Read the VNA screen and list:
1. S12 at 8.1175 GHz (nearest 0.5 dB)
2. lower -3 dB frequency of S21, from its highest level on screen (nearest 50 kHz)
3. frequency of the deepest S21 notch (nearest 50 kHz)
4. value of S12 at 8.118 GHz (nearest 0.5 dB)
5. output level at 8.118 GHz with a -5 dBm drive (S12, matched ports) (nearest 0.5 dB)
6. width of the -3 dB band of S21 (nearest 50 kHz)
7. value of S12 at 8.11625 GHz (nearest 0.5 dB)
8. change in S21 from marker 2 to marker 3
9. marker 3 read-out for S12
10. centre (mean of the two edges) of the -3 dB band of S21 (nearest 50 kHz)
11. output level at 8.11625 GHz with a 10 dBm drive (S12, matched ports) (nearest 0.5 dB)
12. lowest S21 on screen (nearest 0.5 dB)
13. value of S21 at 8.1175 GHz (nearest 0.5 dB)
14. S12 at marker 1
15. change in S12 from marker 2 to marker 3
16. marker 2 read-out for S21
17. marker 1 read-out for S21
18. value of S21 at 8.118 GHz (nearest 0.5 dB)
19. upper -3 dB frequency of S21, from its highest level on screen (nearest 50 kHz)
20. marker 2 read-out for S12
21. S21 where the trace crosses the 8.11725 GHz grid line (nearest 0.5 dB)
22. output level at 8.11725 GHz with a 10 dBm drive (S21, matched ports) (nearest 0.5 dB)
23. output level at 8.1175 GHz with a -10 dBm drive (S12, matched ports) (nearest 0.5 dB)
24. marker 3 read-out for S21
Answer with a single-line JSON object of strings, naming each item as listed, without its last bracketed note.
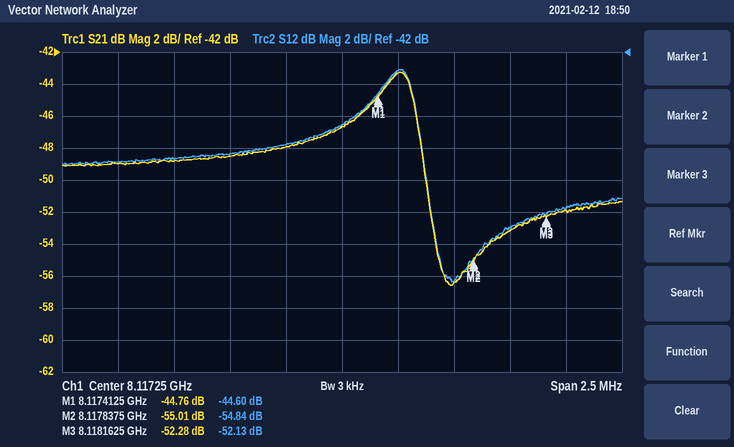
{"S12 at 8.1175 GHz": "-43.0 dB", "lower -3 dB frequency of S21, from its highest level on screen": "8.11730 GHz", "frequency of the deepest S21 notch": "8.11775 GHz", "value of S12 at 8.118 GHz": "-53.0 dB", "output level at 8.118 GHz with a -5 dBm drive (S12, matched ports)": "-58.0 dBm", "width of the -3 dB band of S21": "300 kHz", "value of S12 at 8.11625 GHz": "-49.0 dB", "change in S21 from marker 2 to marker 3": "2.73 dB", "marker 3 read-out for S12": "-52.13 dB", "centre (mean of the two edges) of the -3 dB band of S21": "8.11745 GHz", "output level at 8.11625 GHz with a 10 dBm drive (S12, matched ports)": "-39.0 dBm", "lowest S21 on screen": "-56.5 dB", "value of S21 at 8.1175 GHz": "-43.5 dB", "S12 at marker 1": "-44.60 dB", "change in S12 from marker 2 to marker 3": "2.71 dB", "marker 2 read-out for S21": "-55.01 dB", "marker 1 read-out for S21": "-44.76 dB", "value of S21 at 8.118 GHz": "-53.0 dB", "upper -3 dB frequency of S21, from its highest level on screen": "8.11760 GHz", "marker 2 read-out for S12": "-54.84 dB", "S21 where the trace crosses the 8.11725 GHz grid line": "-46.5 dB", "output level at 8.11725 GHz with a 10 dBm drive (S21, matched ports)": "-36.5 dBm", "output level at 8.1175 GHz with a -10 dBm drive (S12, matched ports)": "-53.0 dBm", "marker 3 read-out for S21": "-52.28 dB"}
